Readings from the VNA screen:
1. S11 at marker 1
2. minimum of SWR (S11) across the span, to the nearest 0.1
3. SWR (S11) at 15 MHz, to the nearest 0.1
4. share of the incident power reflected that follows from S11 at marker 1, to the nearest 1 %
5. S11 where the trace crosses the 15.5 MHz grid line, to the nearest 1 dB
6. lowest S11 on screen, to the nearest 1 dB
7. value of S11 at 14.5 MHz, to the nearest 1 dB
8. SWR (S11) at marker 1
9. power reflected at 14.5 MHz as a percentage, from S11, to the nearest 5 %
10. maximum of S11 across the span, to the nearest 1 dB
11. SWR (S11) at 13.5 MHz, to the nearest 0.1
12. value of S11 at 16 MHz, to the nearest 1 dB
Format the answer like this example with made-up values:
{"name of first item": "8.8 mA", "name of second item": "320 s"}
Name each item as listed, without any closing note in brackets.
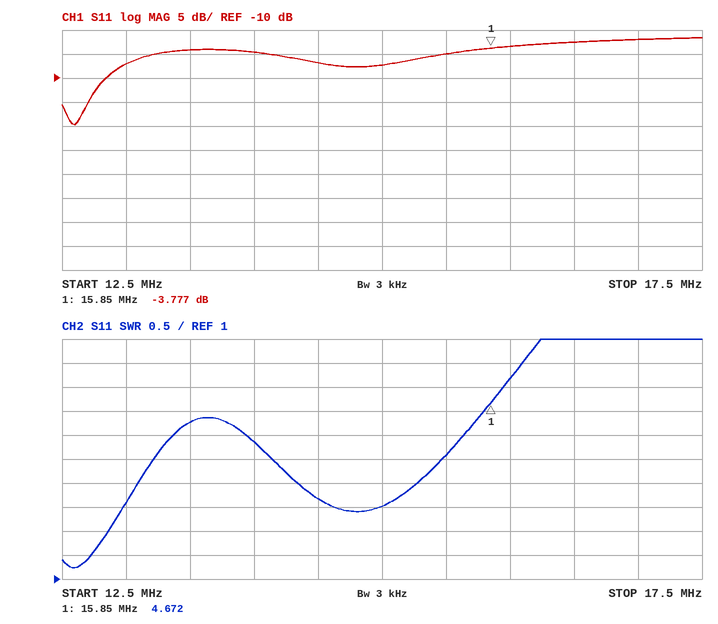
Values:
{"S11 at marker 1": "-3.777 dB", "minimum of SWR (S11) across the span, to the nearest 0.1": "1.2", "SWR (S11) at 15 MHz, to the nearest 0.1": "2.5", "share of the incident power reflected that follows from S11 at marker 1, to the nearest 1 %": "42 %", "S11 where the trace crosses the 15.5 MHz grid line, to the nearest 1 dB": "-5 dB", "lowest S11 on screen, to the nearest 1 dB": "-20 dB", "value of S11 at 14.5 MHz, to the nearest 1 dB": "-7 dB", "SWR (S11) at marker 1": "4.672", "power reflected at 14.5 MHz as a percentage, from S11, to the nearest 5 %": "20 %", "maximum of S11 across the span, to the nearest 1 dB": "-2 dB", "SWR (S11) at 13.5 MHz, to the nearest 0.1": "4.3", "value of S11 at 16 MHz, to the nearest 1 dB": "-3 dB"}
